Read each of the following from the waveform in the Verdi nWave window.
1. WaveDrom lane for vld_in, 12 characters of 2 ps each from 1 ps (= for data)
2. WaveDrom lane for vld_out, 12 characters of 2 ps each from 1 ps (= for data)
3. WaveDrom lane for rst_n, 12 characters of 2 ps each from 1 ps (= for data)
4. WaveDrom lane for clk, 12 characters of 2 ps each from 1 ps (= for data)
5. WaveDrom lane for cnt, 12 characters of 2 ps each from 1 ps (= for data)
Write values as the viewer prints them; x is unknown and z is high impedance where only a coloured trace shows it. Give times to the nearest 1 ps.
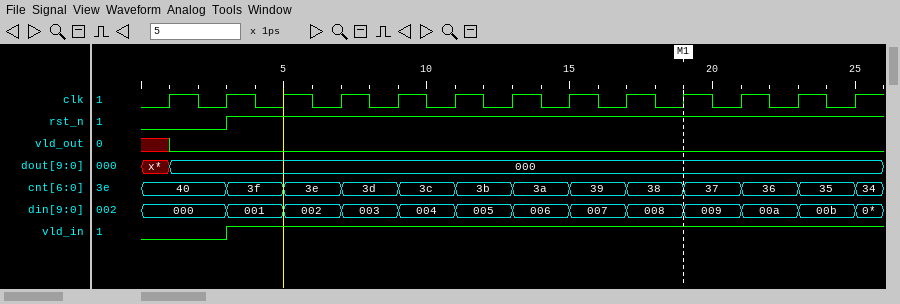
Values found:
{name: 'vld_in', wave: '01..........'}
{name: 'vld_out', wave: '0...........'}
{name: 'rst_n', wave: '01..........'}
{name: 'clk', wave: 'p...........'}
{name: 'cnt', wave: '============', data: '40 3f 3e 3d 3c 3b 3a 39 38 37 36 35'}
